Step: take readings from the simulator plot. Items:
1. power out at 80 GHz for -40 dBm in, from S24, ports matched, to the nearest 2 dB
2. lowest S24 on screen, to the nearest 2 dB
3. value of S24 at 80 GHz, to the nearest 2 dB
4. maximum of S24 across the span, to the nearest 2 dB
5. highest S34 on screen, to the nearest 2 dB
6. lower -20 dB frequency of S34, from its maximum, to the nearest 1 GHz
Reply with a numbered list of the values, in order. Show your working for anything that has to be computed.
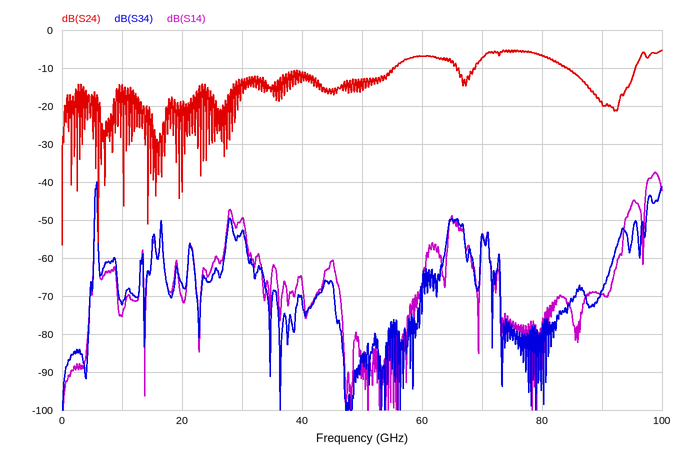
1. -40 dBm + (-6 dB) = -46 dBm
2. -56 dB
3. -6 dB
4. -6 dB
5. -40 dB
6. 5 GHz
